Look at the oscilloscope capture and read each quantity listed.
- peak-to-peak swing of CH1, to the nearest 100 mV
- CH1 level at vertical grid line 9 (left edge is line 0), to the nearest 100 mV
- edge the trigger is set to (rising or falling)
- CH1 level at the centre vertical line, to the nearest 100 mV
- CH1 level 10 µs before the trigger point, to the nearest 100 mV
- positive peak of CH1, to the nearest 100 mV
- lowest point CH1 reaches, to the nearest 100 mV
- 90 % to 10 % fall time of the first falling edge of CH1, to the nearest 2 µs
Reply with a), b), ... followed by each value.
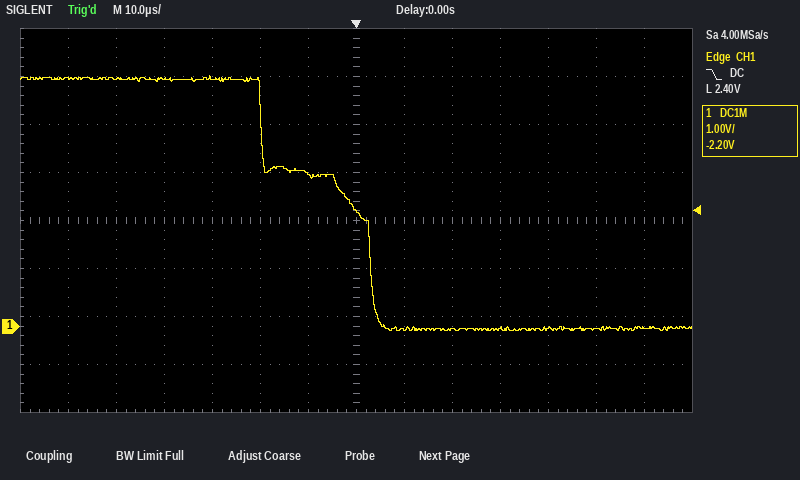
a) 5.3 V
b) -100 mV
c) falling
d) 2.4 V
e) 3.2 V
f) 5.2 V
g) -100 mV
h) 24 µs
